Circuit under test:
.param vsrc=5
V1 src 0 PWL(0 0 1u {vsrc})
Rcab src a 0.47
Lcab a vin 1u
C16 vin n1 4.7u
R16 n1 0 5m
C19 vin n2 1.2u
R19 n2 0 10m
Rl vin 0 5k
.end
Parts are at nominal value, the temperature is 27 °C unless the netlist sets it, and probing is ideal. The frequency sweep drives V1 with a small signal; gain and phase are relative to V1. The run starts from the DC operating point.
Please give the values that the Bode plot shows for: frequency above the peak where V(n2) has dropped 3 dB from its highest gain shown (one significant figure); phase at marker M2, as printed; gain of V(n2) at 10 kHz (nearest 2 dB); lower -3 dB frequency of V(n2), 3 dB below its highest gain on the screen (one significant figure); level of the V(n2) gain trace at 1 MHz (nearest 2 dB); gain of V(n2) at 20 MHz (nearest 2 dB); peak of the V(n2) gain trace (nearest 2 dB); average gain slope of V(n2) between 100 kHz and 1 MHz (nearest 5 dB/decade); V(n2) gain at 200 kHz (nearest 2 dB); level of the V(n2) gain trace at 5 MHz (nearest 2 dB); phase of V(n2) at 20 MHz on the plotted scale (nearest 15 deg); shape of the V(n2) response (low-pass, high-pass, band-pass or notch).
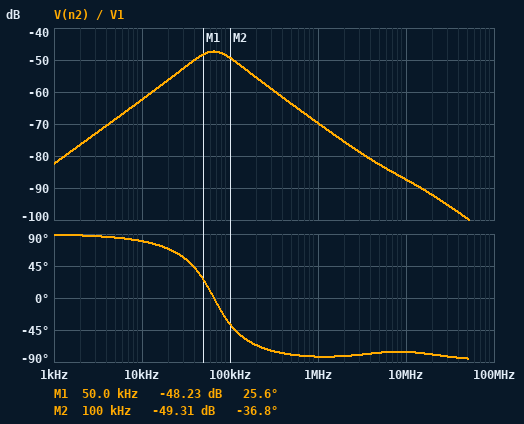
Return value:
100 kHz
-36.8 deg
-62 dB
40 kHz
-70 dB
-92 dB
-48 dB
-20 dB/decade
-56 dB
-82 dB
-75 deg
band-pass
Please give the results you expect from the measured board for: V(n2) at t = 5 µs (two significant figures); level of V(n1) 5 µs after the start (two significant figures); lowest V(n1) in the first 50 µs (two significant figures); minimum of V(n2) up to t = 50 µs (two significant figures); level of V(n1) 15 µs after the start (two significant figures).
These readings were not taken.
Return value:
10 mV
20 mV
-2.7 mV
-1.4 mV
-1.9 mV
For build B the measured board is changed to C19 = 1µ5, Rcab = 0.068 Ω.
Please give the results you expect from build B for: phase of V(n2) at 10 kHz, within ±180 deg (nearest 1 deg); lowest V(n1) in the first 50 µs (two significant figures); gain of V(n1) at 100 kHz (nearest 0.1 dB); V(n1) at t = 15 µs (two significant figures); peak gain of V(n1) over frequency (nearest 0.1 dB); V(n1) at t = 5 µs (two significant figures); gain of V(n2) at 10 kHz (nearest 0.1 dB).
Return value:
88 deg
-31 mV
-40.0 dB
-13 mV
-25.5 dB
39 mV
-60.3 dB
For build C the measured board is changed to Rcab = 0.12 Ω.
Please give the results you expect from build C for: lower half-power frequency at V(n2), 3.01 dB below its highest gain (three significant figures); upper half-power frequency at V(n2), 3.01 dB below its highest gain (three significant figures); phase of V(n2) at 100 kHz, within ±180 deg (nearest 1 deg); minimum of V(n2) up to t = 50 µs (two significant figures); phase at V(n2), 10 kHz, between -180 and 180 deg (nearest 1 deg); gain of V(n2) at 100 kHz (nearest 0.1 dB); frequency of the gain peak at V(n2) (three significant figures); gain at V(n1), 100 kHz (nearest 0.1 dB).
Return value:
56.4 kHz
76.1 kHz
-71 deg
-12 mV
87 deg
-45.4 dB
65.5 kHz
-39.6 dB
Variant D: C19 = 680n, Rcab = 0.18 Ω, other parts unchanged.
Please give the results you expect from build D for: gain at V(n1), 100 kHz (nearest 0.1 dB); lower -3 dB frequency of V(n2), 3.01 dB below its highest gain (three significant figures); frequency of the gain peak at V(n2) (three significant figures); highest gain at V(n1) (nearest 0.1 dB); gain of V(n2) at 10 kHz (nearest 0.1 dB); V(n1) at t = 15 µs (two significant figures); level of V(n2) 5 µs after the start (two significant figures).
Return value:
-38.8 dB
55.5 kHz
68.6 kHz
-32.5 dB
-67.2 dB
-2.4 mV
9.3 mV
